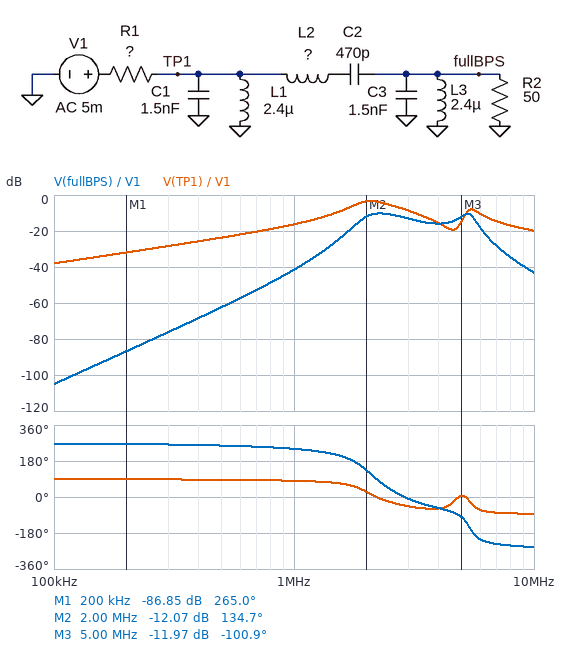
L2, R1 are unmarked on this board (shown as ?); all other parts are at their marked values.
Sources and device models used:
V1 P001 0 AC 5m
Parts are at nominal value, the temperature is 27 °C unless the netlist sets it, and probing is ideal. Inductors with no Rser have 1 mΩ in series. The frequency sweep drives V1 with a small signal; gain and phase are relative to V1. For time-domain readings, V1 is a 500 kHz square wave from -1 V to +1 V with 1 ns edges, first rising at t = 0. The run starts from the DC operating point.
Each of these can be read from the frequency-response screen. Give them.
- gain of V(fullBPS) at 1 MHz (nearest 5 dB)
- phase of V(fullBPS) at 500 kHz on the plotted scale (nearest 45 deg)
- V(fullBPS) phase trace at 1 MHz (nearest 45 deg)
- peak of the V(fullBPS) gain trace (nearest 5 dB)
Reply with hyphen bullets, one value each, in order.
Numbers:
- -40 dB
- 270 deg
- 225 deg
- -10 dB
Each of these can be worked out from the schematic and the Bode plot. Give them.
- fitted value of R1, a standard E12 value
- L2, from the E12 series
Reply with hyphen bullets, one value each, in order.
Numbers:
- 120 Ω
- 3.3 µH
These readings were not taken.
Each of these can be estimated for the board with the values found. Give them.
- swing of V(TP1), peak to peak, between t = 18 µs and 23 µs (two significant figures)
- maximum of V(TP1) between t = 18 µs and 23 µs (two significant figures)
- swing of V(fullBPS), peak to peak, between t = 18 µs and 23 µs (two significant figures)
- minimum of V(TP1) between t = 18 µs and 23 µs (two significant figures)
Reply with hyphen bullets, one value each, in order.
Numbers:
- 840 mV
- 420 mV
- 330 mV
- -420 mV
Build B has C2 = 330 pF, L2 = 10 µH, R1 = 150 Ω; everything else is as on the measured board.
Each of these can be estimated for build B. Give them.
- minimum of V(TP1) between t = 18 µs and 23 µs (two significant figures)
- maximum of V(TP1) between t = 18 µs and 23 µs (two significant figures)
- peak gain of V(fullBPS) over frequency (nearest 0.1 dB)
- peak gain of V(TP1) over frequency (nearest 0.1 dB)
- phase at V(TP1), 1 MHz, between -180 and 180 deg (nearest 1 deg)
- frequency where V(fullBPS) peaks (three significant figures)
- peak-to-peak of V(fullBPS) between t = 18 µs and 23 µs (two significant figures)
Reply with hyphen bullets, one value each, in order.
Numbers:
- -380 mV
- 380 mV
- -10.8 dB
- -4.5 dB
- 83 deg
- 2.15 MHz
- 250 mV
